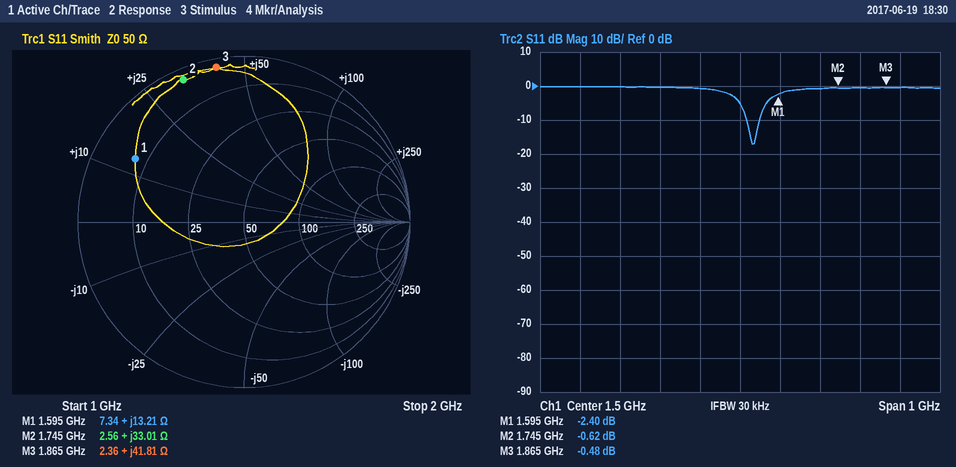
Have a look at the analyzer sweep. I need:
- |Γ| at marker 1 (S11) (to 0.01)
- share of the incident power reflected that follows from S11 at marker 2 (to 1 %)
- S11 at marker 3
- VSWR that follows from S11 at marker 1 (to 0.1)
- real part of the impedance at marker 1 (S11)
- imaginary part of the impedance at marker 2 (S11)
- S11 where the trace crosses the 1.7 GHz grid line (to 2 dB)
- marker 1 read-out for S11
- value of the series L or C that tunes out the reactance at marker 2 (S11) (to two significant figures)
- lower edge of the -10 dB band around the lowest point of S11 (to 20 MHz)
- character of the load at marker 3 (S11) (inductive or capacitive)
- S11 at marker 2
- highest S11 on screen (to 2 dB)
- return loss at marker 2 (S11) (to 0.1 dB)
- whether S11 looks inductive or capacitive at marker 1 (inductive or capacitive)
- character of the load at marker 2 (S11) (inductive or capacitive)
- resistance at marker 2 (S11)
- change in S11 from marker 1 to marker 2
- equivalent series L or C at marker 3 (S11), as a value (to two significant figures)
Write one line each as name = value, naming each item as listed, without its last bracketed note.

|Γ| at marker 1 (S11) = 0.76
share of the incident power reflected that follows from S11 at marker 2 = 87 %
S11 at marker 3 = -0.48 dB
VSWR that follows from S11 at marker 1 = 7.3
real part of the impedance at marker 1 = 7.34 Ω
imaginary part of the impedance at marker 2 = +33.01 Ω
S11 where the trace crosses the 1.7 GHz grid line = 0 dB
marker 1 read-out for S11 = -2.40 dB
value of the series L or C that tunes out the reactance at marker 2 (S11) = 2.8 pF
lower edge of the -10 dB band around the lowest point of S11 = 1.52 GHz
character of the load at marker 3 (S11) = inductive
S11 at marker 2 = -0.62 dB
highest S11 on screen = 0 dB
return loss at marker 2 (S11) = 0.6 dB
whether S11 looks inductive or capacitive at marker 1 = inductive
character of the load at marker 2 (S11) = inductive
resistance at marker 2 = 2.56 Ω
change in S11 from marker 1 to marker 2 = 1.78 dB
equivalent series L or C at marker 3 (S11), as a value = 3.6 nH
